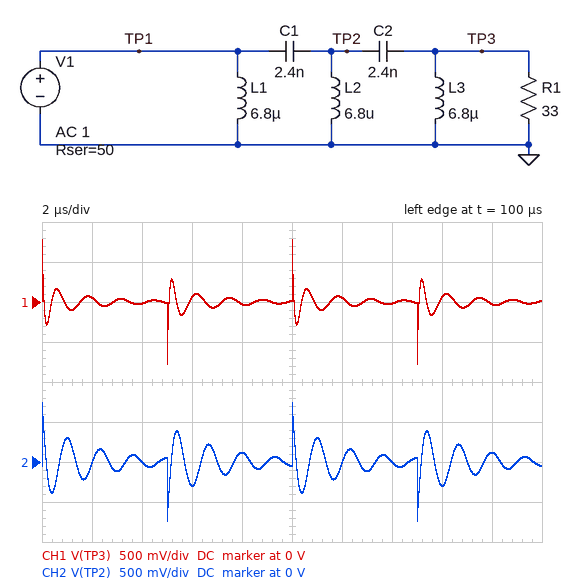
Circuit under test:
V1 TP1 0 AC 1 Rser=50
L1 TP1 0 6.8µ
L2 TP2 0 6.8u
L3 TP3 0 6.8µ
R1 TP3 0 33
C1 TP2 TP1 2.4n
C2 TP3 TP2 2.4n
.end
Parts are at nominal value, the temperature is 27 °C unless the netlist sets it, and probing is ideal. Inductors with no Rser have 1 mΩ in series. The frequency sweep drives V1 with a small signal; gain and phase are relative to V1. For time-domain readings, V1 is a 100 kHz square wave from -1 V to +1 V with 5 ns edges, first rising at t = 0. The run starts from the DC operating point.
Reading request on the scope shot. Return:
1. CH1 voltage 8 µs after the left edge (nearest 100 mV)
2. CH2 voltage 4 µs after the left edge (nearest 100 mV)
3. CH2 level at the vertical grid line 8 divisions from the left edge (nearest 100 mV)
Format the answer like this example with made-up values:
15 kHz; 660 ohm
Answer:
0 V; 0 V; -300 mV
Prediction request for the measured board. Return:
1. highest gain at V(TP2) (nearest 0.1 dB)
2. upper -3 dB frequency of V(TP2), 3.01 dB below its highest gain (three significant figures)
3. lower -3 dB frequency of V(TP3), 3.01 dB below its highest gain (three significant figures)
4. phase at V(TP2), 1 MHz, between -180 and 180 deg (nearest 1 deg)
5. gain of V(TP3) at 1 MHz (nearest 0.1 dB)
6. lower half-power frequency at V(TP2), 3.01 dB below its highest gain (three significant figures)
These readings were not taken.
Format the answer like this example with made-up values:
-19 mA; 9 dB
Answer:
1.6 dB; 889 kHz; 726 kHz; 75 deg; -9.9 dB; 712 kHz
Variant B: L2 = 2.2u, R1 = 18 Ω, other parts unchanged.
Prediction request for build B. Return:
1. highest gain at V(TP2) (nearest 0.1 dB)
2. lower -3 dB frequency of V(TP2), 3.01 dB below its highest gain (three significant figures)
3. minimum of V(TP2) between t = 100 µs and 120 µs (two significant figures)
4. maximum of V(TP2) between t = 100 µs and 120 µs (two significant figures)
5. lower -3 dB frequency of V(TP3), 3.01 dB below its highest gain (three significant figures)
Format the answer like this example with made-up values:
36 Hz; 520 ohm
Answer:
-4.0 dB; 1.08 MHz; -530 mV; 530 mV; 1.28 MHz
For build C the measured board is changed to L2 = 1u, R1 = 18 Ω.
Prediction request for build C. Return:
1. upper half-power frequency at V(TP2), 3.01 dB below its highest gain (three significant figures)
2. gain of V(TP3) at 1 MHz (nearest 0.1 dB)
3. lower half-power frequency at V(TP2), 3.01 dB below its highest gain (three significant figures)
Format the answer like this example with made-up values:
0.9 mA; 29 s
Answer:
9.84 MHz; -30.5 dB; 1.54 MHz
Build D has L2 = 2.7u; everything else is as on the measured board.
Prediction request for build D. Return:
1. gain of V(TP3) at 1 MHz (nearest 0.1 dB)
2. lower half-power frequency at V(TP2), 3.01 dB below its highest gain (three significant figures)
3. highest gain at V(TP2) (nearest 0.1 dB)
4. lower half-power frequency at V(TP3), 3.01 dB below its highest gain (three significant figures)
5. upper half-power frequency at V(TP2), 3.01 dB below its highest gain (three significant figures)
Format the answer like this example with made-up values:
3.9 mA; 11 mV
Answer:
-12.5 dB; 963 kHz; -4.2 dB; 1.05 MHz; 2.75 MHz
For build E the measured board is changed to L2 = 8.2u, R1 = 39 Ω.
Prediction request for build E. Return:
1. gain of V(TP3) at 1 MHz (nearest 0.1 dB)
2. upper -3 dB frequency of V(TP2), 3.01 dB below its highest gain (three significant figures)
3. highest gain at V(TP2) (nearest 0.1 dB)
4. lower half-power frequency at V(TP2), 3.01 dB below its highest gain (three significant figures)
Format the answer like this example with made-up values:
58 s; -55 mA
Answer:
-10.1 dB; 784 kHz; 2.8 dB; 662 kHz
